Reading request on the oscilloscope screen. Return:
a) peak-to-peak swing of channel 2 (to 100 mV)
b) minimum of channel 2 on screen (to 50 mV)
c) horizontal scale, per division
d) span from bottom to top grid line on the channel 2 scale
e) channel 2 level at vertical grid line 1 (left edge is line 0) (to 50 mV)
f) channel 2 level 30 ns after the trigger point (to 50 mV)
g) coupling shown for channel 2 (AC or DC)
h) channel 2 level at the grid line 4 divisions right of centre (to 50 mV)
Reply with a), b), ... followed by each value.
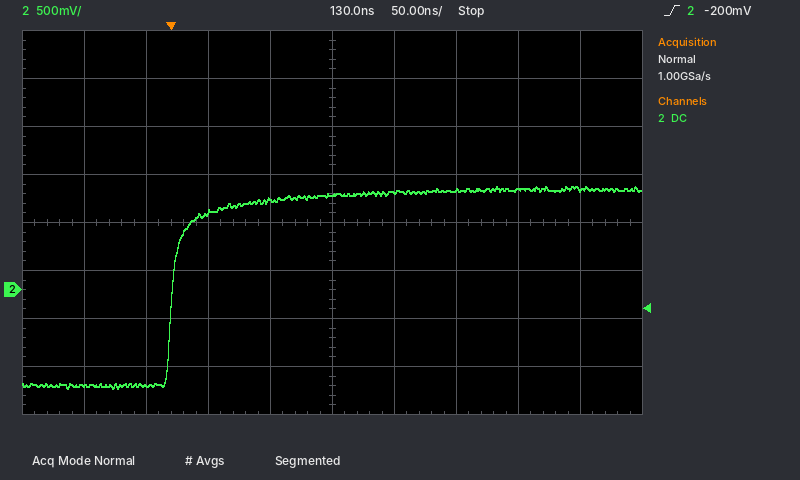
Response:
a) 2.10 V
b) -1.05 V
c) 50 ns
d) 4 V
e) -1.00 V
f) 800 mV
g) DC
h) 1.05 V
